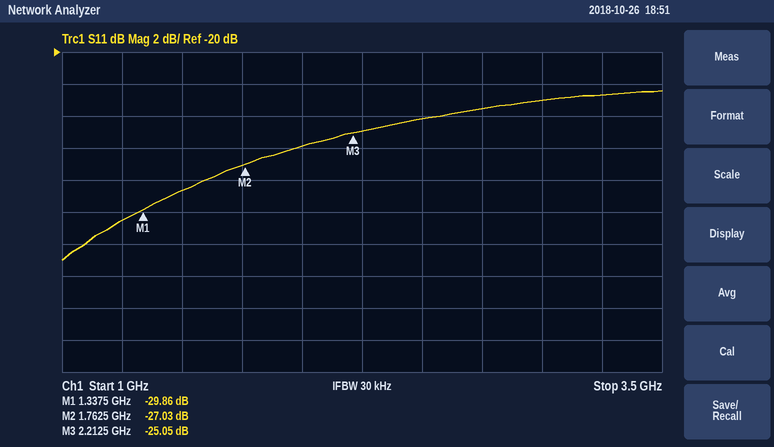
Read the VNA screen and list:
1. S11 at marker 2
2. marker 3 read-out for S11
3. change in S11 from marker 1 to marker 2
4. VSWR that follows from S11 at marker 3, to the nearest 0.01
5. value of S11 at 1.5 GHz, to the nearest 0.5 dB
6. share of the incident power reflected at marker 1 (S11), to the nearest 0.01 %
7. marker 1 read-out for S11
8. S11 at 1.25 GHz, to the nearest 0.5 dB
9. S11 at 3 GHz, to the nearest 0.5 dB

-27.03 dB
-25.05 dB
2.83 dB
1.12
-28.5 dB
0.10 %
-29.86 dB
-30.5 dB
-23.0 dB
